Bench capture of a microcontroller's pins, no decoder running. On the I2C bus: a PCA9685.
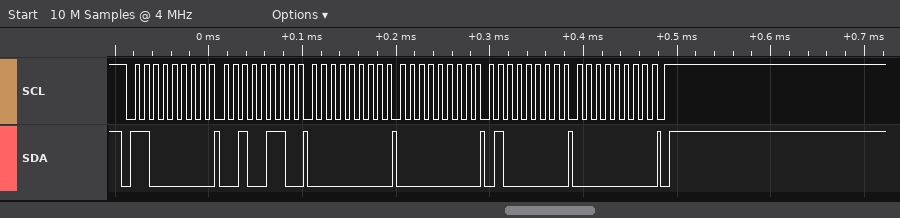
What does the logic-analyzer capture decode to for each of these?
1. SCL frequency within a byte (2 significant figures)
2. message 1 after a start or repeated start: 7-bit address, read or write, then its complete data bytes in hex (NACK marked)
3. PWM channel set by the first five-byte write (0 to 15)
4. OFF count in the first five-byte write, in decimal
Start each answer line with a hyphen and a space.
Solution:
- 100 kHz
- 0x60 write: 26 00 00 40 00
- 8
- 64
